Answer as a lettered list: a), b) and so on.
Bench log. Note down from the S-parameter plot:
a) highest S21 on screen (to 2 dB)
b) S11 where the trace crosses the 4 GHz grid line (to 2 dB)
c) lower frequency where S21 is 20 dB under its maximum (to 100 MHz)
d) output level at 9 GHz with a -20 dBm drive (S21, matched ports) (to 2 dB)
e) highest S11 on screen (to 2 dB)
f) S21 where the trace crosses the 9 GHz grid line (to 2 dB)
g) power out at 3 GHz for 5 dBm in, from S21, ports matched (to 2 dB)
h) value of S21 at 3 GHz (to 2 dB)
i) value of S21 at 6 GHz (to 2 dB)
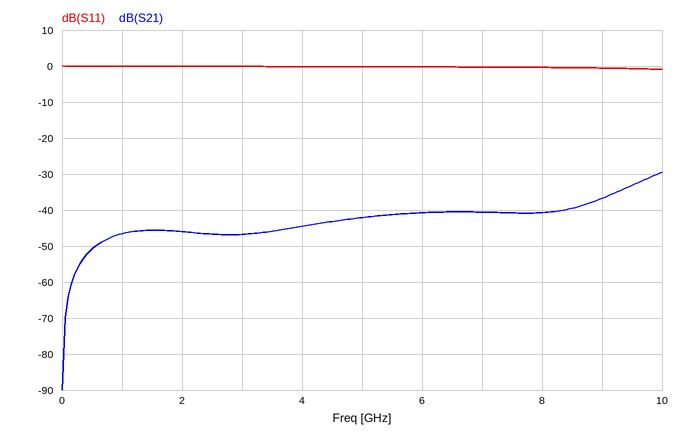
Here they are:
a) -30 dB
b) 0 dB
c) 600 MHz
d) -56 dBm
e) 0 dB
f) -36 dB
g) -42 dBm
h) -46 dB
i) -40 dB
